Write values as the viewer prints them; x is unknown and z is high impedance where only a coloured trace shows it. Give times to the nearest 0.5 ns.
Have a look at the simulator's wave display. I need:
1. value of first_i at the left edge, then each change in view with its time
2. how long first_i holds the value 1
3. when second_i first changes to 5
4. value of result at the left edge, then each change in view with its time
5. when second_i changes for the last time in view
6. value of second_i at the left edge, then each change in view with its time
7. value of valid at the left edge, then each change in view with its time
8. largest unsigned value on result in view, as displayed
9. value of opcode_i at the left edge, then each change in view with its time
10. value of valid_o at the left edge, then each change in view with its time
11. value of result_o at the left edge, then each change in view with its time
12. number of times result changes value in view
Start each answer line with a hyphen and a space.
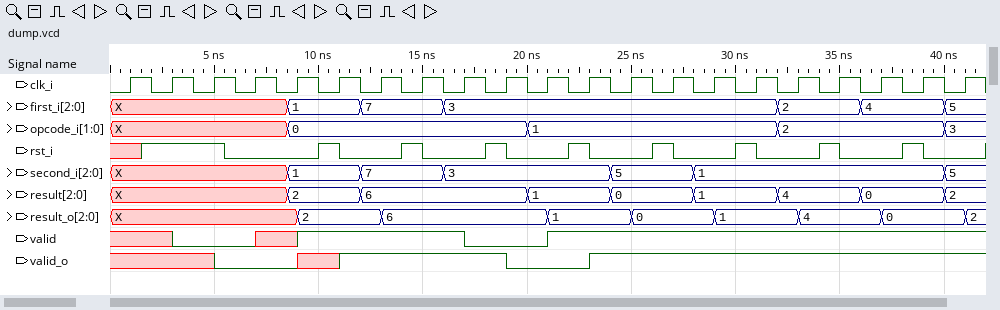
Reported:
- X, 1 at 8.5 ns, 7 at 12 ns, 3 at 16 ns, 2 at 32 ns, 4 at 36 ns, 5 at 40 ns
- 3.5 ns
- 24 ns
- X, 2 at 8.5 ns, 6 at 12 ns, 1 at 20 ns, 0 at 24 ns, 1 at 28 ns, 4 at 32 ns, 0 at 36 ns, 2 at 40 ns
- 40 ns
- X, 1 at 8.5 ns, 7 at 12 ns, 3 at 16 ns, 5 at 24 ns, 1 at 28 ns, 5 at 40 ns
- x, 0 at 3 ns, x at 7 ns, 1 at 9 ns, 0 at 17 ns, 1 at 21 ns
- 6
- X, 0 at 8.5 ns, 1 at 20 ns, 2 at 32 ns, 3 at 40 ns
- x, 0 at 5 ns, x at 9 ns, 1 at 11 ns, 0 at 19 ns, 1 at 23 ns
- X, 2 at 9 ns, 6 at 13 ns, 1 at 21 ns, 0 at 25 ns, 1 at 29 ns, 4 at 33 ns, 0 at 37 ns, 2 at 41 ns
- 8
